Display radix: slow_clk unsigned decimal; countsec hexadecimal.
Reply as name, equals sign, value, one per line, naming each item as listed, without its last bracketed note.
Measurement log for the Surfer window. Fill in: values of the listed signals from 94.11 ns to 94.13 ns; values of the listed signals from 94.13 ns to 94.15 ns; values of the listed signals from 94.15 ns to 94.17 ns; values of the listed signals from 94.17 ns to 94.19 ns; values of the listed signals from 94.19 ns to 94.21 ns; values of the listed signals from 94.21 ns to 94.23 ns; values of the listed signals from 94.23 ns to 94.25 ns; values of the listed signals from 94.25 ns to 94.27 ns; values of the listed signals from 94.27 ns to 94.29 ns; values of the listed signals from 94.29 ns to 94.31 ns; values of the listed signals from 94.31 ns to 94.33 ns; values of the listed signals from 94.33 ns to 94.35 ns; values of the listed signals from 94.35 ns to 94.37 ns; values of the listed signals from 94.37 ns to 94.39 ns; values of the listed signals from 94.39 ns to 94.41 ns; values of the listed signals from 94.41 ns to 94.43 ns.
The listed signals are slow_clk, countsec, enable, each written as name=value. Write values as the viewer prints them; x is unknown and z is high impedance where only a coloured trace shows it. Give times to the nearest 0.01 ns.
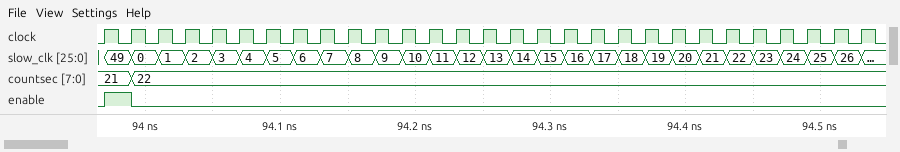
values of the listed signals from 94.11 ns to 94.13 ns = slow_clk=6, countsec=22, enable=0
values of the listed signals from 94.13 ns to 94.15 ns = slow_clk=7, countsec=22, enable=0
values of the listed signals from 94.15 ns to 94.17 ns = slow_clk=8, countsec=22, enable=0
values of the listed signals from 94.17 ns to 94.19 ns = slow_clk=9, countsec=22, enable=0
values of the listed signals from 94.19 ns to 94.21 ns = slow_clk=10, countsec=22, enable=0
values of the listed signals from 94.21 ns to 94.23 ns = slow_clk=11, countsec=22, enable=0
values of the listed signals from 94.23 ns to 94.25 ns = slow_clk=12, countsec=22, enable=0
values of the listed signals from 94.25 ns to 94.27 ns = slow_clk=13, countsec=22, enable=0
values of the listed signals from 94.27 ns to 94.29 ns = slow_clk=14, countsec=22, enable=0
values of the listed signals from 94.29 ns to 94.31 ns = slow_clk=15, countsec=22, enable=0
values of the listed signals from 94.31 ns to 94.33 ns = slow_clk=16, countsec=22, enable=0
values of the listed signals from 94.33 ns to 94.35 ns = slow_clk=17, countsec=22, enable=0
values of the listed signals from 94.35 ns to 94.37 ns = slow_clk=18, countsec=22, enable=0
values of the listed signals from 94.37 ns to 94.39 ns = slow_clk=19, countsec=22, enable=0
values of the listed signals from 94.39 ns to 94.41 ns = slow_clk=20, countsec=22, enable=0
values of the listed signals from 94.41 ns to 94.43 ns = slow_clk=21, countsec=22, enable=0
